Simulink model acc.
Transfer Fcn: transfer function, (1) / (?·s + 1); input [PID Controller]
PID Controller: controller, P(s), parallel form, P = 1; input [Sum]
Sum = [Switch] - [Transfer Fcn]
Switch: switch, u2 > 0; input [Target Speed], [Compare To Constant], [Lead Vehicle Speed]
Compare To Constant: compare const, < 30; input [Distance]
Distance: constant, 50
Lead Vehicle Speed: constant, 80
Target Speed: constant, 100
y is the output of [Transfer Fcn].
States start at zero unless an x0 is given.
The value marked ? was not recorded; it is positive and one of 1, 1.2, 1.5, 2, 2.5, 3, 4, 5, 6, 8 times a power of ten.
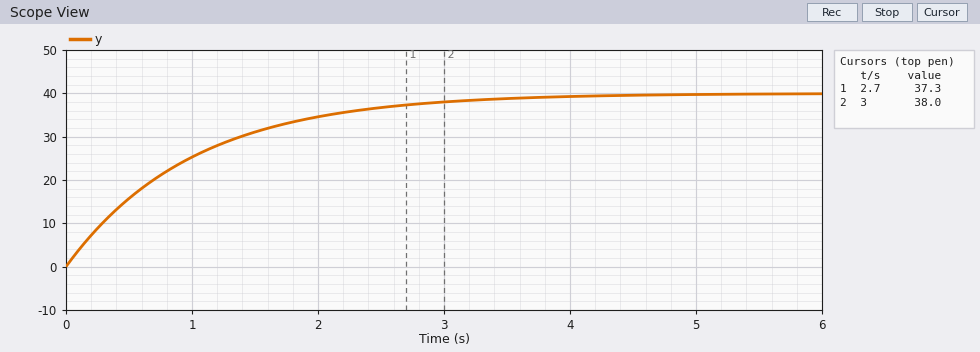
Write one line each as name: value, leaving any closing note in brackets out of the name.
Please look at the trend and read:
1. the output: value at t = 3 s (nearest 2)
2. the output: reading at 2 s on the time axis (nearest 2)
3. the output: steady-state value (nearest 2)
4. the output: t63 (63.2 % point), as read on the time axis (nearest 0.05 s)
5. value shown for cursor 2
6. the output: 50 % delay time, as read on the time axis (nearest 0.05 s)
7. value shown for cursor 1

the output: value at t = 3 s: 38
the output: reading at 2 s on the time axis: 34
the output: steady-state value: 40
the output: t63 (63.2 % point), as read on the time axis: 1.00 s
value shown for cursor 2: 38.0
the output: 50 % delay time, as read on the time axis: 0.70 s
value shown for cursor 1: 37.3
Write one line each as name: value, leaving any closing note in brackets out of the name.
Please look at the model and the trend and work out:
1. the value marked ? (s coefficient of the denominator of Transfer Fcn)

the value marked ?: 2
